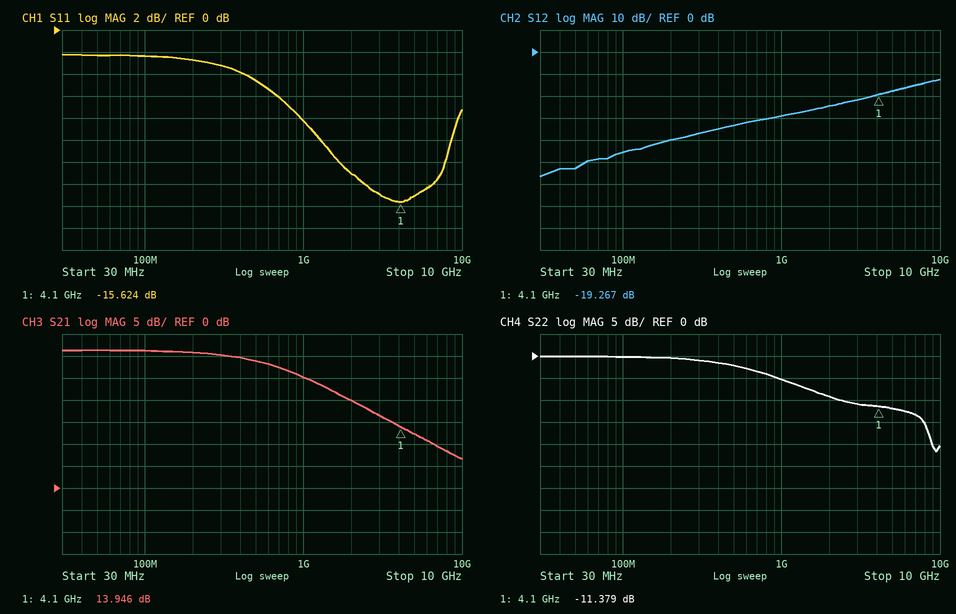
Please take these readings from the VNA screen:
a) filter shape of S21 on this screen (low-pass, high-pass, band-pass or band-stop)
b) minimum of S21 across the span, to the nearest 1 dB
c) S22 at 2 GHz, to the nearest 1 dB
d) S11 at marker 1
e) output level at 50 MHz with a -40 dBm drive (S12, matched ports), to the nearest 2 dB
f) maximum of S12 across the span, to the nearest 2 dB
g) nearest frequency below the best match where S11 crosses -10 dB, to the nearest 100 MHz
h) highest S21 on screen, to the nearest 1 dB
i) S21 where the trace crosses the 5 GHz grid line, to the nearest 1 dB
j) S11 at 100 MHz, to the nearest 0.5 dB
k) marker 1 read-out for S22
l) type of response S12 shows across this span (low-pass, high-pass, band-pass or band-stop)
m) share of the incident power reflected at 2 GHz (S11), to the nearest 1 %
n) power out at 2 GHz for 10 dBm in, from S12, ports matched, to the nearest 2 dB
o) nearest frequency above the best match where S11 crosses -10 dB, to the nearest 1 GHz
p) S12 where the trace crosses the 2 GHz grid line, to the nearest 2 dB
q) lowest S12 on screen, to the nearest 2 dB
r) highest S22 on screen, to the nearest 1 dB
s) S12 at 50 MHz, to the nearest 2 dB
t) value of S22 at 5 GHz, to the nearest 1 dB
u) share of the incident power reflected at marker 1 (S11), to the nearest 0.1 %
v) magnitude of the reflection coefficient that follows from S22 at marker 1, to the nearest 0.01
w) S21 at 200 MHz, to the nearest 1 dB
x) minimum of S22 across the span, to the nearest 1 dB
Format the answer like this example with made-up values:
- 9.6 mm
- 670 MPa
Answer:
- low-pass
- 7 dB
- -9 dB
- -15.624 dB
- -92 dBm
- -12 dB
- 1.3 GHz
- 31 dB
- 12 dB
- -2.5 dB
- -11.379 dB
- high-pass
- 5 %
- -14 dBm
- 9 GHz
- -24 dB
- -56 dB
- 0 dB
- -52 dB
- -12 dB
- 2.7 %
- 0.27
- 31 dB
- -22 dB
